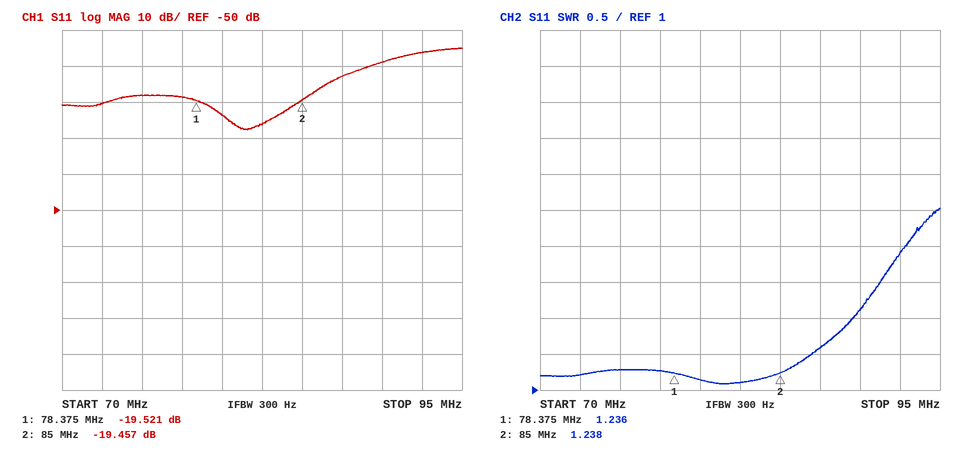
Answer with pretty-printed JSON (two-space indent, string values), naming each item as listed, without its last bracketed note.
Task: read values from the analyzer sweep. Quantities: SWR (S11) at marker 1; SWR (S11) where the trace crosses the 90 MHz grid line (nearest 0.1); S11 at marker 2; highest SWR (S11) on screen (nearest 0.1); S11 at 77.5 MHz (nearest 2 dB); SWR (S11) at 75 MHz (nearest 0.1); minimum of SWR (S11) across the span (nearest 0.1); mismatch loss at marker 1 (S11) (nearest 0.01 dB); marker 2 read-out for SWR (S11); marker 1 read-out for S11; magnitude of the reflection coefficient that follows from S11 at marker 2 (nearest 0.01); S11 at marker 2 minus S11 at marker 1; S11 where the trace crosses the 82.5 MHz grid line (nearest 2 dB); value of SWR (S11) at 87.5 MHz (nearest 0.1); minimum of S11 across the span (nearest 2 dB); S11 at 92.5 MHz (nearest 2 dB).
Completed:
{
  "SWR (S11) at marker 1": "1.236",
  "SWR (S11) where the trace crosses the 90 MHz grid line": "2.1",
  "S11 at marker 2": "-19.457 dB",
  "highest SWR (S11) on screen": "3.5",
  "S11 at 77.5 MHz": "-18 dB",
  "SWR (S11) at 75 MHz": "1.3",
  "minimum of SWR (S11) across the span": "1.1",
  "mismatch loss at marker 1 (S11)": "0.05 dB",
  "marker 2 read-out for SWR": "1.238",
  "marker 1 read-out for S11": "-19.521 dB",
  "magnitude of the reflection coefficient that follows from S11 at marker 2": "0.11",
  "S11 at marker 2 minus S11 at marker 1": "0.064 dB",
  "S11 where the trace crosses the 82.5 MHz grid line": "-26 dB",
  "value of SWR (S11) at 87.5 MHz": "1.6",
  "minimum of S11 across the span": "-28 dB",
  "S11 at 92.5 MHz": "-6 dB"
}
